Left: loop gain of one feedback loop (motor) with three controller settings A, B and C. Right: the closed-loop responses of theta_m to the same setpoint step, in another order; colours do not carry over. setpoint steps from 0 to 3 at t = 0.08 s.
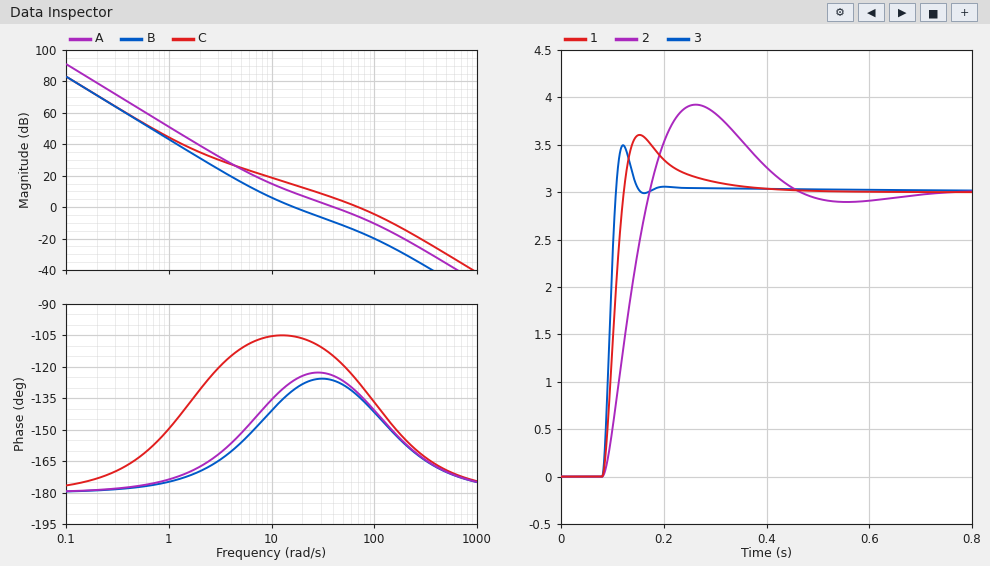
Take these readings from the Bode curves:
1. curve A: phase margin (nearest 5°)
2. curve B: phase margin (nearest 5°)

55°
50°
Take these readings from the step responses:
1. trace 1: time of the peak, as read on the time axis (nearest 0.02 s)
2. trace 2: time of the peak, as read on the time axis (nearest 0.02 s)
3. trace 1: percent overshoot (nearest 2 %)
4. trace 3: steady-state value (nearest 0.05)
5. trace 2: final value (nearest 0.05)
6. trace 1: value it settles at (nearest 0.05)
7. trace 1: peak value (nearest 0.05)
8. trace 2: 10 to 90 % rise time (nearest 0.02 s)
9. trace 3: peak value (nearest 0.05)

0.16 s
0.26 s
20 %
3.00
3.00
3.00
3.60
0.06 s
3.50
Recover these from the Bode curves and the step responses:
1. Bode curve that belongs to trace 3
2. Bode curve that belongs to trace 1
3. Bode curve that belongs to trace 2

C
A
B
